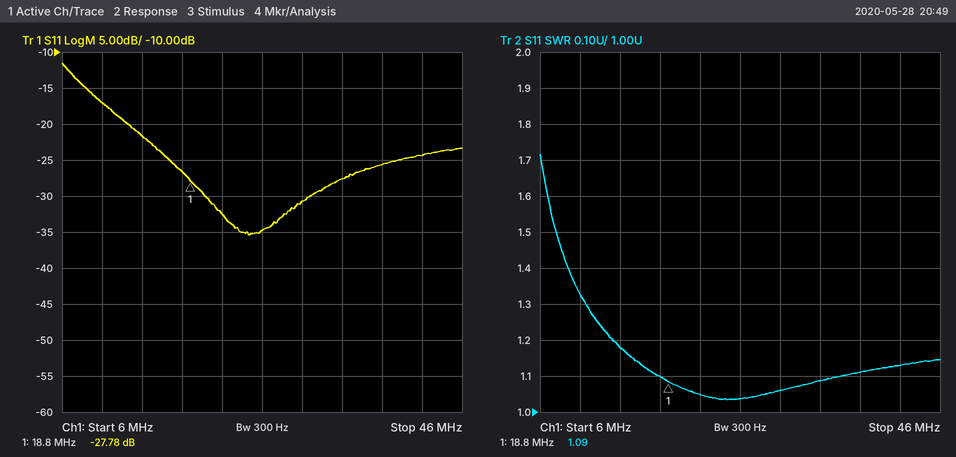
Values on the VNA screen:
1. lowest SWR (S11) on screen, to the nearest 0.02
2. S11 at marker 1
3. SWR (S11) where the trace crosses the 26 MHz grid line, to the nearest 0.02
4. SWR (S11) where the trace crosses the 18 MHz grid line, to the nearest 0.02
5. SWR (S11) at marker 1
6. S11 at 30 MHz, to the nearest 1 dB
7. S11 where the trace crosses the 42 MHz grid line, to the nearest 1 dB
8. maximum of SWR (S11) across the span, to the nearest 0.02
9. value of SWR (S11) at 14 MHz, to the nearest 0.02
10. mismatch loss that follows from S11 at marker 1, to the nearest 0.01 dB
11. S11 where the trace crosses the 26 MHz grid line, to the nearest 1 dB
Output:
1.04
-27.78 dB
1.04
1.10
1.09
-31 dB
-24 dB
1.72
1.18
0.01 dB
-35 dB
